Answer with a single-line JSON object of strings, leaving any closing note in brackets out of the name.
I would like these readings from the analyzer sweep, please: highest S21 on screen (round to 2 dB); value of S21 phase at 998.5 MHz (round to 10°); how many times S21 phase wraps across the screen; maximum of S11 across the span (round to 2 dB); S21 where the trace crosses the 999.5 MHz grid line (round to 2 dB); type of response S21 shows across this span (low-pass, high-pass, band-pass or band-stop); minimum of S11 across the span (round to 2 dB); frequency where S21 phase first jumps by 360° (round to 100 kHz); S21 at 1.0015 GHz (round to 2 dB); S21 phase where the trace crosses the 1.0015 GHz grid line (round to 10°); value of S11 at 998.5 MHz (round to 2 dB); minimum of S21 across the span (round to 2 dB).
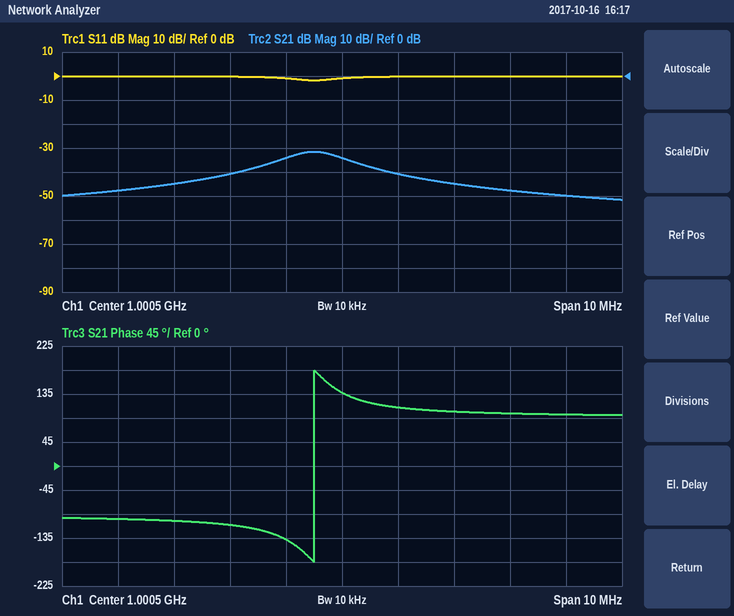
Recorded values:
{"highest S21 on screen": "-32 dB", "value of S21 phase at 998.5 MHz": "-110°", "how many times S21 phase wraps across the screen": "1", "maximum of S11 across the span": "0 dB", "S21 where the trace crosses the 999.5 MHz grid line": "-34 dB", "type of response S21 shows across this span": "band-pass", "minimum of S11 across the span": "-2 dB", "frequency where S21 phase first jumps by 360°": "1.0000 GHz", "S21 at 1.0015 GHz": "-40 dB", "S21 phase where the trace crosses the 1.0015 GHz grid line": "110°", "value of S11 at 998.5 MHz": "0 dB", "minimum of S21 across the span": "-52 dB"}
